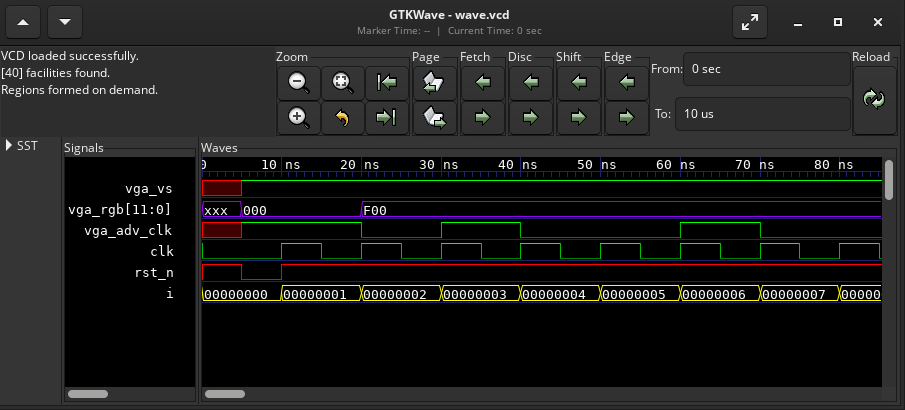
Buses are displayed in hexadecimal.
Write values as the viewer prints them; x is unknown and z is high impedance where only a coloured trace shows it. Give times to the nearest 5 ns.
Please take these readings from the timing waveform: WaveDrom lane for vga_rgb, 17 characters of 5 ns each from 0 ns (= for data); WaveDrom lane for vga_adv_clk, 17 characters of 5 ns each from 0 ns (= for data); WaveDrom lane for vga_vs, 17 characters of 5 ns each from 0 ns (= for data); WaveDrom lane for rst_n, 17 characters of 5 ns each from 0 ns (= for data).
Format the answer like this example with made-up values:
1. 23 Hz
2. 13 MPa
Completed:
1. {name: 'vga_rgb', wave: 'x=..=............', data: '000 F00'}
2. {name: 'vga_adv_clk', wave: 'x1..0.1.0...1.0..'}
3. {name: 'vga_vs', wave: 'x1...............'}
4. {name: 'rst_n', wave: '101..............'}
